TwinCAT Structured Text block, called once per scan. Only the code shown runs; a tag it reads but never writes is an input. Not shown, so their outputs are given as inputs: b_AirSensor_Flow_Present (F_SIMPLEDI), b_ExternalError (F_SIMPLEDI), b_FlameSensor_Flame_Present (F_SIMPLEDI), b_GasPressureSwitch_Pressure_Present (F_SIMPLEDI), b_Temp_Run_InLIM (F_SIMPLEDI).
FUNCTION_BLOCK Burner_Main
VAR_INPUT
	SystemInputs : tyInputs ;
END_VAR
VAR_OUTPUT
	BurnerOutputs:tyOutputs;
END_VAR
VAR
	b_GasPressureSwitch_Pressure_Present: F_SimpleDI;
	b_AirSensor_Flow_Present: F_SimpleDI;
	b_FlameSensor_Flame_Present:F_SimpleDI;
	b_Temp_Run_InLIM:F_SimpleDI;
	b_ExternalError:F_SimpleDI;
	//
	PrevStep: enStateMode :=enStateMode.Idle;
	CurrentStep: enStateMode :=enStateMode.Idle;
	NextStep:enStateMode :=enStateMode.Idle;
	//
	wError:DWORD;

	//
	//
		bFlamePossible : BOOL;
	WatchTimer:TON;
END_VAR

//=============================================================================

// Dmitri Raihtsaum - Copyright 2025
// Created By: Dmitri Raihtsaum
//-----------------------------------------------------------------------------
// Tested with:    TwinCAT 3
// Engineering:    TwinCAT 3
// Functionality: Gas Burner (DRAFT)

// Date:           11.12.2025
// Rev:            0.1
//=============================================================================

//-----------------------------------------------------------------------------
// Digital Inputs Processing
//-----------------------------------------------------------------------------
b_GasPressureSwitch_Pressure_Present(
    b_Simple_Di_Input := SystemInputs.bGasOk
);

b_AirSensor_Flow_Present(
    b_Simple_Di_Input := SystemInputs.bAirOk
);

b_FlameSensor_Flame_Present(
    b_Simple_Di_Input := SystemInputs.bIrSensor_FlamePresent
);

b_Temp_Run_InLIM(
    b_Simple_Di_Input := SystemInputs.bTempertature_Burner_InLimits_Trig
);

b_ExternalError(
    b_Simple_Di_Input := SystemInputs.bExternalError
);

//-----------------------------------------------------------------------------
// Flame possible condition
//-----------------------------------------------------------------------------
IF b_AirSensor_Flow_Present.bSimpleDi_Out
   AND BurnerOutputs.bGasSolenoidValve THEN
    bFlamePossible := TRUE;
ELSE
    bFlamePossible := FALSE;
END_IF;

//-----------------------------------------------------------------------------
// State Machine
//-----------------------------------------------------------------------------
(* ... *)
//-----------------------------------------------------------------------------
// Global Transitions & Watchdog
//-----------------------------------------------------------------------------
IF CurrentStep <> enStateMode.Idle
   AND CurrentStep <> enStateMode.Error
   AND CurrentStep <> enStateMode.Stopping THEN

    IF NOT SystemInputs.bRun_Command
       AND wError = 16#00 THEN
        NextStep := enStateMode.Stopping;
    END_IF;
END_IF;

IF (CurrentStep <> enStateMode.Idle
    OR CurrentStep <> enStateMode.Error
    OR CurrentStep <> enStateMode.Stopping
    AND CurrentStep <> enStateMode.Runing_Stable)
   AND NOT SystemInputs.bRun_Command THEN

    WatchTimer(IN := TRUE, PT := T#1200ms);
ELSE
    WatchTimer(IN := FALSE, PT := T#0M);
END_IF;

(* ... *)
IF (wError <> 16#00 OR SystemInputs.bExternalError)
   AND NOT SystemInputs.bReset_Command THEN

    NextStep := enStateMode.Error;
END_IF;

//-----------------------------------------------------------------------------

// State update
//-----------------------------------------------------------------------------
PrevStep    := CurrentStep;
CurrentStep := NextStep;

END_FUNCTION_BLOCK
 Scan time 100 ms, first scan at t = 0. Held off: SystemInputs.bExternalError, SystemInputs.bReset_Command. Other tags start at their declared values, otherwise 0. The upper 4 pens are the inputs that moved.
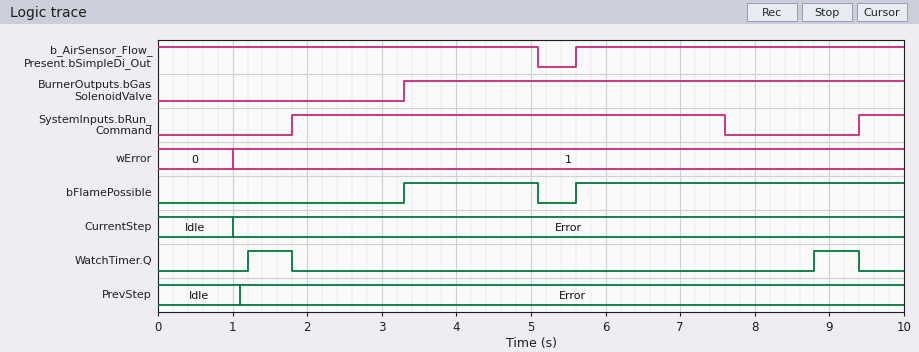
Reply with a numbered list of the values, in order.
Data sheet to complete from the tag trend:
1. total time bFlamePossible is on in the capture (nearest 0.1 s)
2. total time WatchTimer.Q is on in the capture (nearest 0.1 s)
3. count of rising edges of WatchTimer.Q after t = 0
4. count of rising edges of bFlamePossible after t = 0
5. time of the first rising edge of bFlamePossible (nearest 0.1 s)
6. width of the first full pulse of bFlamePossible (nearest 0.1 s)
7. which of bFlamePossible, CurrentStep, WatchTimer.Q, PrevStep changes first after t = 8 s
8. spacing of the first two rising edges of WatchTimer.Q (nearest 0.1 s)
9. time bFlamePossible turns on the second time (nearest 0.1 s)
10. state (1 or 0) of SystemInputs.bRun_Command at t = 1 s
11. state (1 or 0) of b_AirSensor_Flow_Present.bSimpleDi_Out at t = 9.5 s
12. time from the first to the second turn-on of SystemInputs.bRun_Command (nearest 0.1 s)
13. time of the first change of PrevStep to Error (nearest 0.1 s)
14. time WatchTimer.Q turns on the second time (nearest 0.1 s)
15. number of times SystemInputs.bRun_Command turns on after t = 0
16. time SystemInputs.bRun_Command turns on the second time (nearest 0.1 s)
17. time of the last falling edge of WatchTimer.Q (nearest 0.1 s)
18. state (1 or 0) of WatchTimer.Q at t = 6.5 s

1. 6.2 s
2. 1.2 s
3. 2
4. 2
5. 3.3 s
6. 1.8 s
7. WatchTimer.Q
8. 7.6 s
9. 5.6 s
10. 0
11. 1
12. 7.6 s
13. 1.1 s
14. 8.8 s
15. 2
16. 9.4 s
17. 9.4 s
18. 0
